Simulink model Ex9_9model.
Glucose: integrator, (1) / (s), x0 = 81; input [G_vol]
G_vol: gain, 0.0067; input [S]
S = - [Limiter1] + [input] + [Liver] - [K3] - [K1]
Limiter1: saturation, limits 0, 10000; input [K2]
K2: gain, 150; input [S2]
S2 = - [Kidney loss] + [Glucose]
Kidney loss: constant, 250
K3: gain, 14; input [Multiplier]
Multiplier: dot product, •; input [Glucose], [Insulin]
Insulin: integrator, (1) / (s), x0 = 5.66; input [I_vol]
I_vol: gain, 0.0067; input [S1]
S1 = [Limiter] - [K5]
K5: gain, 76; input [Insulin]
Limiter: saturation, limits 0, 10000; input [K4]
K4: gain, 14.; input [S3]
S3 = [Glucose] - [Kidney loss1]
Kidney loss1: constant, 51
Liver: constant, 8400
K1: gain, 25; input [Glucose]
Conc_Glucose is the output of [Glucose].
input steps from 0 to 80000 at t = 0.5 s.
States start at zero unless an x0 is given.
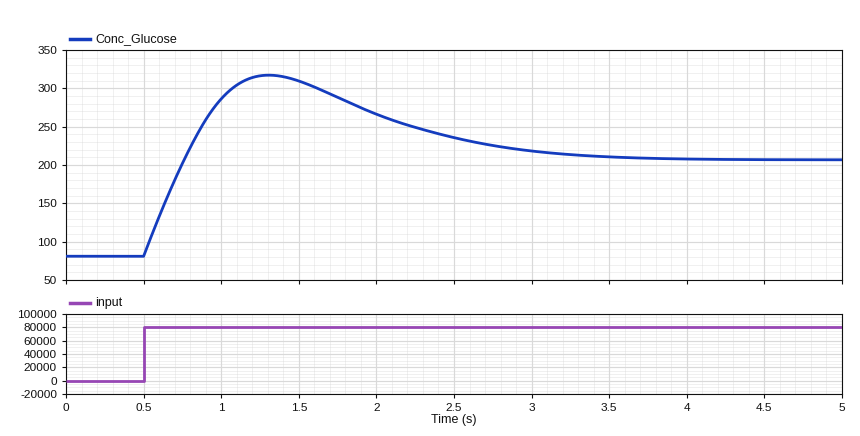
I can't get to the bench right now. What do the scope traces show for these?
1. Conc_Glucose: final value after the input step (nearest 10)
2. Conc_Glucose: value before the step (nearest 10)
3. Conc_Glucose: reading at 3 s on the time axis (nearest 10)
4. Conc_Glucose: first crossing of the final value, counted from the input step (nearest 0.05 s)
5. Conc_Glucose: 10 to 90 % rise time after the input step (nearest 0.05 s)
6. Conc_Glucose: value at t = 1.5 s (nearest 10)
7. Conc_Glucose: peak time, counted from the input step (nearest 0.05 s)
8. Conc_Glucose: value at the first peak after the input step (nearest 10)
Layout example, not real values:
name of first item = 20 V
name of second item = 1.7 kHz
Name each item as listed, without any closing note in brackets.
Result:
Conc_Glucose: final value after the input step = 210
Conc_Glucose: value before the step = 80
Conc_Glucose: reading at 3 s on the time axis = 220
Conc_Glucose: first crossing of the final value, counted from the input step = 0.25 s
Conc_Glucose: 10 to 90 % rise time after the input step = 0.20 s
Conc_Glucose: value at t = 1.5 s = 310
Conc_Glucose: peak time, counted from the input step = 0.80 s
Conc_Glucose: value at the first peak after the input step = 320
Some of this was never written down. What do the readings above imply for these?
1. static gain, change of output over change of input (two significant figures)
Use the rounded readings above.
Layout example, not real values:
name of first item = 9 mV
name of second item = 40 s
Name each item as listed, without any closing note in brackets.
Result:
static gain, change of output over change of input = 0.0016
